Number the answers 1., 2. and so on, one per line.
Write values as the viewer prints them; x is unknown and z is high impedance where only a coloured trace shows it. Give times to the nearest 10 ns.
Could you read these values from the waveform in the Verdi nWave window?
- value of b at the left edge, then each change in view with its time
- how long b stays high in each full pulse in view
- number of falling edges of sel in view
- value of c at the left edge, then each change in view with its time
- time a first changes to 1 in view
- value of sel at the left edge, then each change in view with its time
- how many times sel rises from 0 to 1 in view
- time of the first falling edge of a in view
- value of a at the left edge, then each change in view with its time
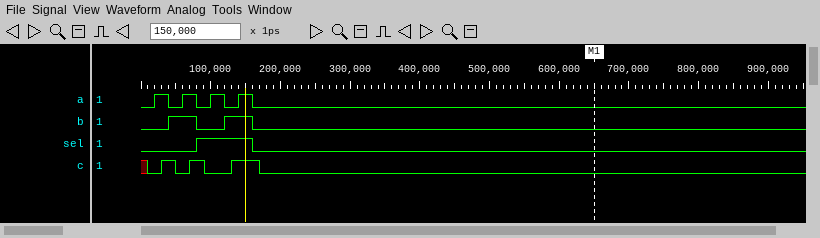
1. 0, 1 at 40 ns, 0 at 80 ns, 1 at 120 ns, 0 at 160 ns
2. 40 ns, 40 ns
3. 1
4. x, 0 at 10 ns, 1 at 30 ns, 0 at 50 ns, 1 at 70 ns, 0 at 90 ns, 1 at 130 ns, 0 at 170 ns
5. 20 ns
6. 0, 1 at 80 ns, 0 at 160 ns
7. 1
8. 40 ns
9. 0, 1 at 20 ns, 0 at 40 ns, 1 at 60 ns, 0 at 80 ns, 1 at 100 ns, 0 at 120 ns, 1 at 140 ns, 0 at 160 ns
